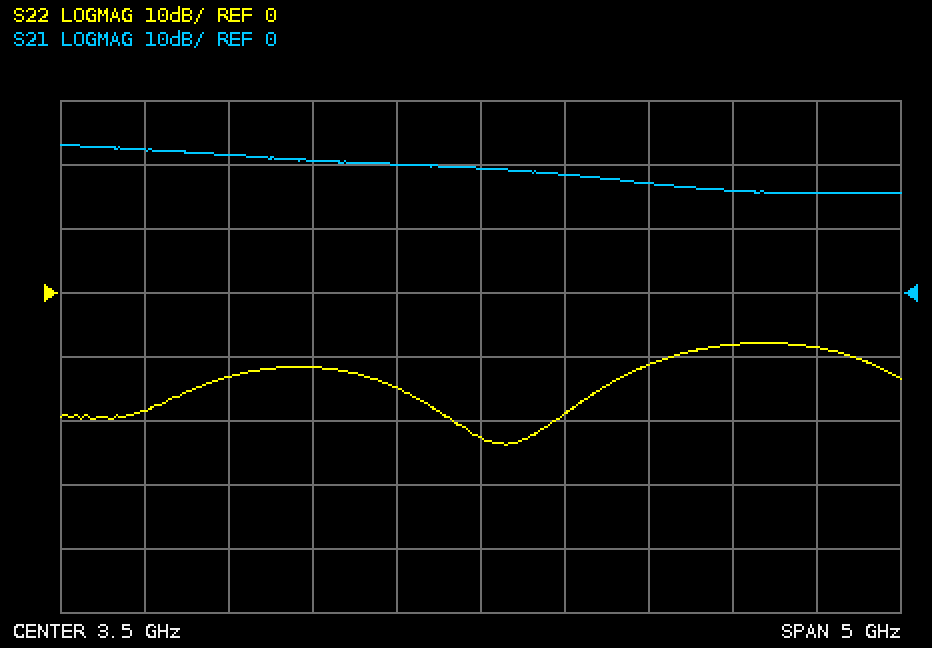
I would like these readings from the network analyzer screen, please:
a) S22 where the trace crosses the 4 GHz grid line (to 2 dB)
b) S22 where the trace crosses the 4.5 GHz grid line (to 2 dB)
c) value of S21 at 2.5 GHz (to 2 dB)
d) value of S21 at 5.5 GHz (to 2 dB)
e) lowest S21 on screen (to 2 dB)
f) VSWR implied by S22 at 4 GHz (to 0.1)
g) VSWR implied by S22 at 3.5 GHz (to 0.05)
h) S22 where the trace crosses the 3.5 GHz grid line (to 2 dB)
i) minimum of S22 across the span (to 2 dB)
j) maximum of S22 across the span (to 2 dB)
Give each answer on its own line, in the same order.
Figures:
-18 dB
-12 dB
20 dB
16 dB
16 dB
1.3
1.15
-22 dB
-24 dB
-8 dB
